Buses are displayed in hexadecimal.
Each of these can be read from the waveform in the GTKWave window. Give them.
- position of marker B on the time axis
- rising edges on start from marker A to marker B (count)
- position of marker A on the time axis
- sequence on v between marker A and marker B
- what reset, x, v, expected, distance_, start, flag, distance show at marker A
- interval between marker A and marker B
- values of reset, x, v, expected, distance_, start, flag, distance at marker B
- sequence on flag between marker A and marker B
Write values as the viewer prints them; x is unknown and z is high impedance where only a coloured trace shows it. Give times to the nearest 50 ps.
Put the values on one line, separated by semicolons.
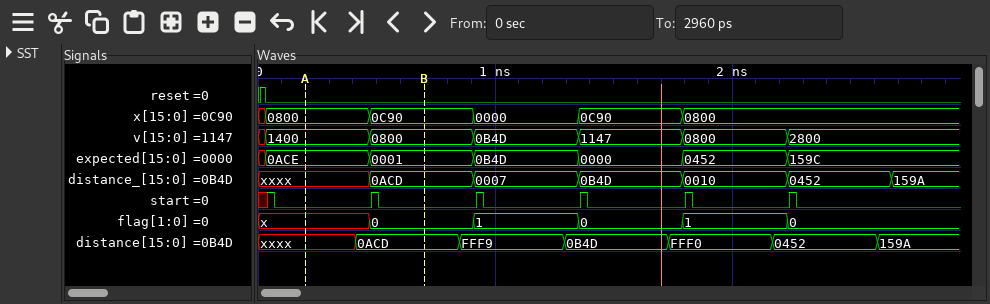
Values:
700 ps; 1; 200 ps; 1400, 0800; reset=0, x=0800, v=1400, expected=0ACE, distance_=xxxx, start=0, flag=x, distance=xxxx; 500 ps; reset=0, x=0C90, v=0800, expected=0001, distance_=0ACD, start=0, flag=0, distance=0ACD; x, 0
